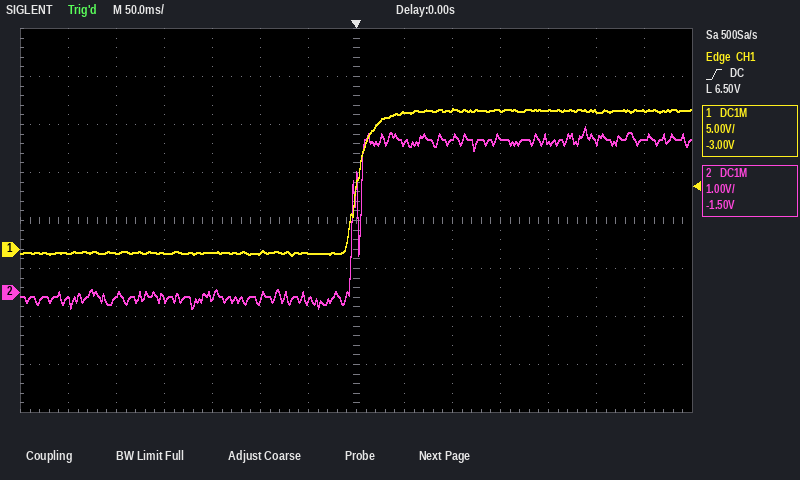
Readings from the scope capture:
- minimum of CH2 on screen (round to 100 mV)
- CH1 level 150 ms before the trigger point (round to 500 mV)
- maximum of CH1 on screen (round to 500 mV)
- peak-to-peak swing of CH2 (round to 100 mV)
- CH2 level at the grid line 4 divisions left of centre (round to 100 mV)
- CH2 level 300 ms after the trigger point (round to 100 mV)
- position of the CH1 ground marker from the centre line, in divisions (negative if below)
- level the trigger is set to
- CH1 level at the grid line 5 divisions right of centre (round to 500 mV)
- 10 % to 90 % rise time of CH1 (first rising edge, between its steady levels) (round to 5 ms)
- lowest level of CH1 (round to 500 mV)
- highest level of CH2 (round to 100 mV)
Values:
-300 mV
-500 mV
14.5 V
3.8 V
-100 mV
3.2 V
-0.6 div
6.50 V
14.5 V
30 ms
-500 mV
3.5 V
